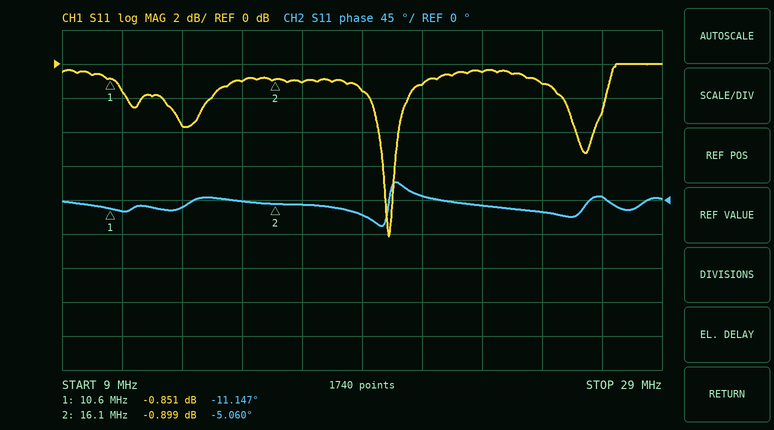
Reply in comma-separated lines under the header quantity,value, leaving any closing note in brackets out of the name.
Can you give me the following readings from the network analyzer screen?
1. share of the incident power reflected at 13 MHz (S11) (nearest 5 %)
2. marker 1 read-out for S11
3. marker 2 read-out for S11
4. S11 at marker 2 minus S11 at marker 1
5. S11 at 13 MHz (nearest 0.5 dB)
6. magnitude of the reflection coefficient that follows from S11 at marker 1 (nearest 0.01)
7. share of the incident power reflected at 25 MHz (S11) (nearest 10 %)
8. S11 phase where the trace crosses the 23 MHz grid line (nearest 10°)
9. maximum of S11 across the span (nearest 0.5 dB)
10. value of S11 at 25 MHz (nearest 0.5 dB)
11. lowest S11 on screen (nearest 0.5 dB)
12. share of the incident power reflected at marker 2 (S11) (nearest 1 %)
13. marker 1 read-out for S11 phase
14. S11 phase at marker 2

quantity,value
share of the incident power reflected at 13 MHz (S11),45 %
marker 1 read-out for S11,-0.851 dB
marker 2 read-out for S11,-0.899 dB
S11 at marker 2 minus S11 at marker 1,-0.048 dB
S11 at 13 MHz,-3.5 dB
magnitude of the reflection coefficient that follows from S11 at marker 1,0.91
share of the incident power reflected at 25 MHz (S11),80 %
S11 phase where the trace crosses the 23 MHz grid line,-10°
maximum of S11 across the span,0.0 dB
value of S11 at 25 MHz,-1.0 dB
lowest S11 on screen,-10.0 dB
share of the incident power reflected at marker 2 (S11),81 %
marker 1 read-out for S11 phase,-11.147°
S11 phase at marker 2,-5.060°
